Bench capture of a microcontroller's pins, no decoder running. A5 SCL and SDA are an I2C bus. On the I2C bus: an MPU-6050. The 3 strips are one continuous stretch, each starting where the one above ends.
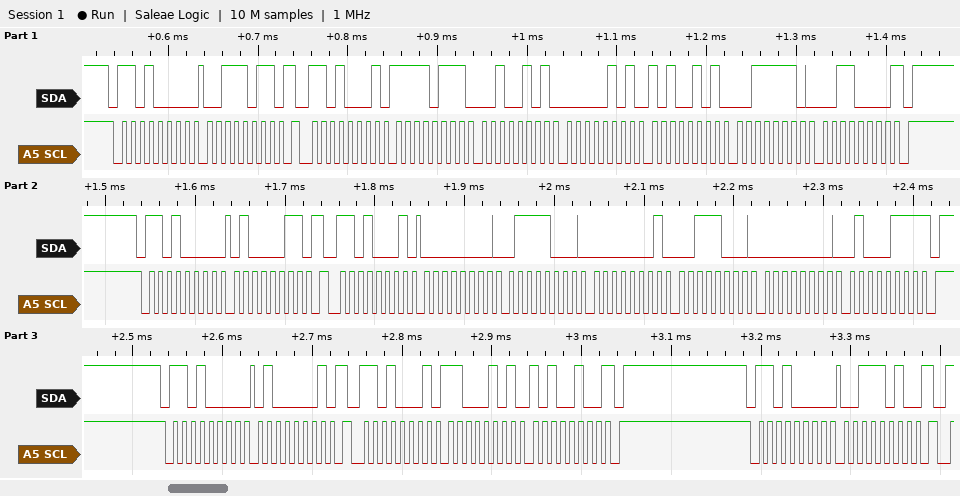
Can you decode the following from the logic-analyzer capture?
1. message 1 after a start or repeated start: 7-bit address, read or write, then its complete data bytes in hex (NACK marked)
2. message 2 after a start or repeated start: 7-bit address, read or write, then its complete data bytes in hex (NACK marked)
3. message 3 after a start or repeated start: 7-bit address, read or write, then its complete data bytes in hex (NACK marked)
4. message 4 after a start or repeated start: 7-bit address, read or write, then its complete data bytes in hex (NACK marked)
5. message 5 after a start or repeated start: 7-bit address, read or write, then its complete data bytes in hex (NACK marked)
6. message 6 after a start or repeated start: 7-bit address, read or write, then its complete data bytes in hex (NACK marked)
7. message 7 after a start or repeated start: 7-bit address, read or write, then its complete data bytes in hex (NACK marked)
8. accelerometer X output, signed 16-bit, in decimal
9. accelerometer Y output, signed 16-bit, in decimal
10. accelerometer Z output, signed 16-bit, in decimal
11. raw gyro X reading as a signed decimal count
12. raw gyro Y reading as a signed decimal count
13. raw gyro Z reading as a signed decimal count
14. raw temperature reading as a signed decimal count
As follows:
0x68 write: 3B
0x68 read: F7 25 05 A5 3E 30 NACK
0x68 write: 43
0x68 read: 00 78 01 38 00 47 NACK
0x68 write: 41
0x68 read: C5 A4 NACK
0x68 write: 3A
-2267
1445
15920
120
312
71
-14940
